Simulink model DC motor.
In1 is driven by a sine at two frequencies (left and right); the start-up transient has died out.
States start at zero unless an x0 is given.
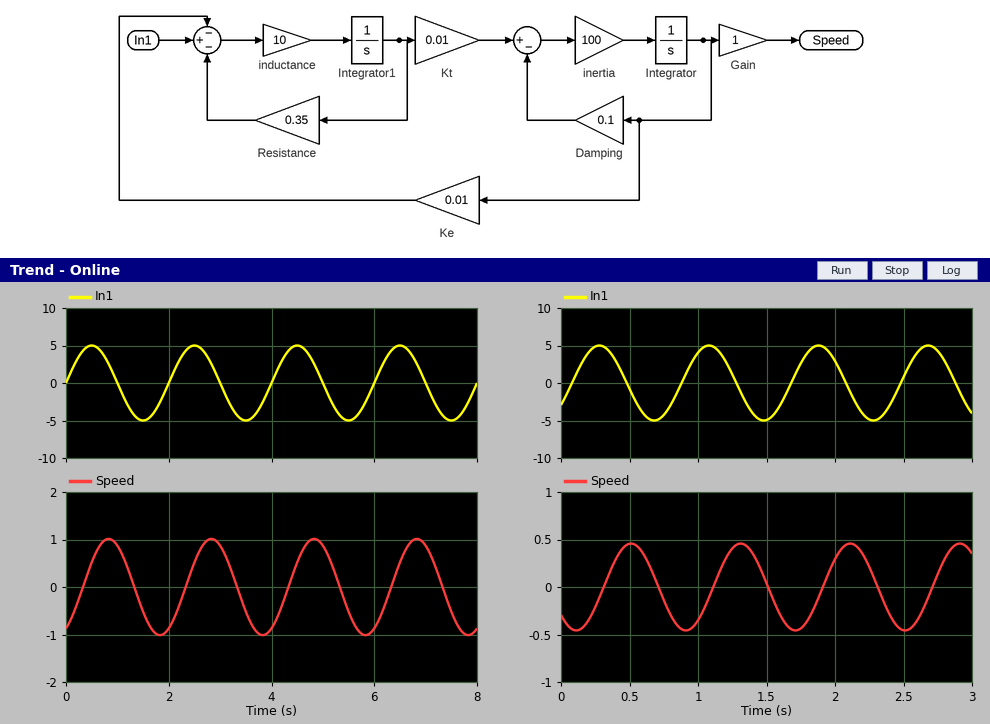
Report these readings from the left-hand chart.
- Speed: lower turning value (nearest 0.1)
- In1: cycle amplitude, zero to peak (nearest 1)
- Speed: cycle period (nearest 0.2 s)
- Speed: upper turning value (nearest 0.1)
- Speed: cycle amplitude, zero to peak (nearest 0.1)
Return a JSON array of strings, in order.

["-1.0", "5", "2.0 s", "1.0", "1.0"]
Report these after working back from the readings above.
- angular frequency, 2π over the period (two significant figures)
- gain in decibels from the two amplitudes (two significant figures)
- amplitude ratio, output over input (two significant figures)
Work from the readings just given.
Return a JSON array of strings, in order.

["3.1 rad/s", "-14 dB", "0.20"]
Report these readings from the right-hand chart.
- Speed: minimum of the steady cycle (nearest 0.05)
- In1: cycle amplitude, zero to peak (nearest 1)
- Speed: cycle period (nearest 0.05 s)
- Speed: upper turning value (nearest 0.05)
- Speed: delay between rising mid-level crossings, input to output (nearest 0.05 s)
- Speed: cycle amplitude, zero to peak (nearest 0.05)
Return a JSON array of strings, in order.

["-0.45", "5", "0.80 s", "0.45", "0.25 s", "0.45"]
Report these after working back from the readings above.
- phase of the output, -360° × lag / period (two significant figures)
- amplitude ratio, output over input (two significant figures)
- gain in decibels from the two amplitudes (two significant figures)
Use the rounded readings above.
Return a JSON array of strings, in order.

["-110°", "0.090", "-21 dB"]
